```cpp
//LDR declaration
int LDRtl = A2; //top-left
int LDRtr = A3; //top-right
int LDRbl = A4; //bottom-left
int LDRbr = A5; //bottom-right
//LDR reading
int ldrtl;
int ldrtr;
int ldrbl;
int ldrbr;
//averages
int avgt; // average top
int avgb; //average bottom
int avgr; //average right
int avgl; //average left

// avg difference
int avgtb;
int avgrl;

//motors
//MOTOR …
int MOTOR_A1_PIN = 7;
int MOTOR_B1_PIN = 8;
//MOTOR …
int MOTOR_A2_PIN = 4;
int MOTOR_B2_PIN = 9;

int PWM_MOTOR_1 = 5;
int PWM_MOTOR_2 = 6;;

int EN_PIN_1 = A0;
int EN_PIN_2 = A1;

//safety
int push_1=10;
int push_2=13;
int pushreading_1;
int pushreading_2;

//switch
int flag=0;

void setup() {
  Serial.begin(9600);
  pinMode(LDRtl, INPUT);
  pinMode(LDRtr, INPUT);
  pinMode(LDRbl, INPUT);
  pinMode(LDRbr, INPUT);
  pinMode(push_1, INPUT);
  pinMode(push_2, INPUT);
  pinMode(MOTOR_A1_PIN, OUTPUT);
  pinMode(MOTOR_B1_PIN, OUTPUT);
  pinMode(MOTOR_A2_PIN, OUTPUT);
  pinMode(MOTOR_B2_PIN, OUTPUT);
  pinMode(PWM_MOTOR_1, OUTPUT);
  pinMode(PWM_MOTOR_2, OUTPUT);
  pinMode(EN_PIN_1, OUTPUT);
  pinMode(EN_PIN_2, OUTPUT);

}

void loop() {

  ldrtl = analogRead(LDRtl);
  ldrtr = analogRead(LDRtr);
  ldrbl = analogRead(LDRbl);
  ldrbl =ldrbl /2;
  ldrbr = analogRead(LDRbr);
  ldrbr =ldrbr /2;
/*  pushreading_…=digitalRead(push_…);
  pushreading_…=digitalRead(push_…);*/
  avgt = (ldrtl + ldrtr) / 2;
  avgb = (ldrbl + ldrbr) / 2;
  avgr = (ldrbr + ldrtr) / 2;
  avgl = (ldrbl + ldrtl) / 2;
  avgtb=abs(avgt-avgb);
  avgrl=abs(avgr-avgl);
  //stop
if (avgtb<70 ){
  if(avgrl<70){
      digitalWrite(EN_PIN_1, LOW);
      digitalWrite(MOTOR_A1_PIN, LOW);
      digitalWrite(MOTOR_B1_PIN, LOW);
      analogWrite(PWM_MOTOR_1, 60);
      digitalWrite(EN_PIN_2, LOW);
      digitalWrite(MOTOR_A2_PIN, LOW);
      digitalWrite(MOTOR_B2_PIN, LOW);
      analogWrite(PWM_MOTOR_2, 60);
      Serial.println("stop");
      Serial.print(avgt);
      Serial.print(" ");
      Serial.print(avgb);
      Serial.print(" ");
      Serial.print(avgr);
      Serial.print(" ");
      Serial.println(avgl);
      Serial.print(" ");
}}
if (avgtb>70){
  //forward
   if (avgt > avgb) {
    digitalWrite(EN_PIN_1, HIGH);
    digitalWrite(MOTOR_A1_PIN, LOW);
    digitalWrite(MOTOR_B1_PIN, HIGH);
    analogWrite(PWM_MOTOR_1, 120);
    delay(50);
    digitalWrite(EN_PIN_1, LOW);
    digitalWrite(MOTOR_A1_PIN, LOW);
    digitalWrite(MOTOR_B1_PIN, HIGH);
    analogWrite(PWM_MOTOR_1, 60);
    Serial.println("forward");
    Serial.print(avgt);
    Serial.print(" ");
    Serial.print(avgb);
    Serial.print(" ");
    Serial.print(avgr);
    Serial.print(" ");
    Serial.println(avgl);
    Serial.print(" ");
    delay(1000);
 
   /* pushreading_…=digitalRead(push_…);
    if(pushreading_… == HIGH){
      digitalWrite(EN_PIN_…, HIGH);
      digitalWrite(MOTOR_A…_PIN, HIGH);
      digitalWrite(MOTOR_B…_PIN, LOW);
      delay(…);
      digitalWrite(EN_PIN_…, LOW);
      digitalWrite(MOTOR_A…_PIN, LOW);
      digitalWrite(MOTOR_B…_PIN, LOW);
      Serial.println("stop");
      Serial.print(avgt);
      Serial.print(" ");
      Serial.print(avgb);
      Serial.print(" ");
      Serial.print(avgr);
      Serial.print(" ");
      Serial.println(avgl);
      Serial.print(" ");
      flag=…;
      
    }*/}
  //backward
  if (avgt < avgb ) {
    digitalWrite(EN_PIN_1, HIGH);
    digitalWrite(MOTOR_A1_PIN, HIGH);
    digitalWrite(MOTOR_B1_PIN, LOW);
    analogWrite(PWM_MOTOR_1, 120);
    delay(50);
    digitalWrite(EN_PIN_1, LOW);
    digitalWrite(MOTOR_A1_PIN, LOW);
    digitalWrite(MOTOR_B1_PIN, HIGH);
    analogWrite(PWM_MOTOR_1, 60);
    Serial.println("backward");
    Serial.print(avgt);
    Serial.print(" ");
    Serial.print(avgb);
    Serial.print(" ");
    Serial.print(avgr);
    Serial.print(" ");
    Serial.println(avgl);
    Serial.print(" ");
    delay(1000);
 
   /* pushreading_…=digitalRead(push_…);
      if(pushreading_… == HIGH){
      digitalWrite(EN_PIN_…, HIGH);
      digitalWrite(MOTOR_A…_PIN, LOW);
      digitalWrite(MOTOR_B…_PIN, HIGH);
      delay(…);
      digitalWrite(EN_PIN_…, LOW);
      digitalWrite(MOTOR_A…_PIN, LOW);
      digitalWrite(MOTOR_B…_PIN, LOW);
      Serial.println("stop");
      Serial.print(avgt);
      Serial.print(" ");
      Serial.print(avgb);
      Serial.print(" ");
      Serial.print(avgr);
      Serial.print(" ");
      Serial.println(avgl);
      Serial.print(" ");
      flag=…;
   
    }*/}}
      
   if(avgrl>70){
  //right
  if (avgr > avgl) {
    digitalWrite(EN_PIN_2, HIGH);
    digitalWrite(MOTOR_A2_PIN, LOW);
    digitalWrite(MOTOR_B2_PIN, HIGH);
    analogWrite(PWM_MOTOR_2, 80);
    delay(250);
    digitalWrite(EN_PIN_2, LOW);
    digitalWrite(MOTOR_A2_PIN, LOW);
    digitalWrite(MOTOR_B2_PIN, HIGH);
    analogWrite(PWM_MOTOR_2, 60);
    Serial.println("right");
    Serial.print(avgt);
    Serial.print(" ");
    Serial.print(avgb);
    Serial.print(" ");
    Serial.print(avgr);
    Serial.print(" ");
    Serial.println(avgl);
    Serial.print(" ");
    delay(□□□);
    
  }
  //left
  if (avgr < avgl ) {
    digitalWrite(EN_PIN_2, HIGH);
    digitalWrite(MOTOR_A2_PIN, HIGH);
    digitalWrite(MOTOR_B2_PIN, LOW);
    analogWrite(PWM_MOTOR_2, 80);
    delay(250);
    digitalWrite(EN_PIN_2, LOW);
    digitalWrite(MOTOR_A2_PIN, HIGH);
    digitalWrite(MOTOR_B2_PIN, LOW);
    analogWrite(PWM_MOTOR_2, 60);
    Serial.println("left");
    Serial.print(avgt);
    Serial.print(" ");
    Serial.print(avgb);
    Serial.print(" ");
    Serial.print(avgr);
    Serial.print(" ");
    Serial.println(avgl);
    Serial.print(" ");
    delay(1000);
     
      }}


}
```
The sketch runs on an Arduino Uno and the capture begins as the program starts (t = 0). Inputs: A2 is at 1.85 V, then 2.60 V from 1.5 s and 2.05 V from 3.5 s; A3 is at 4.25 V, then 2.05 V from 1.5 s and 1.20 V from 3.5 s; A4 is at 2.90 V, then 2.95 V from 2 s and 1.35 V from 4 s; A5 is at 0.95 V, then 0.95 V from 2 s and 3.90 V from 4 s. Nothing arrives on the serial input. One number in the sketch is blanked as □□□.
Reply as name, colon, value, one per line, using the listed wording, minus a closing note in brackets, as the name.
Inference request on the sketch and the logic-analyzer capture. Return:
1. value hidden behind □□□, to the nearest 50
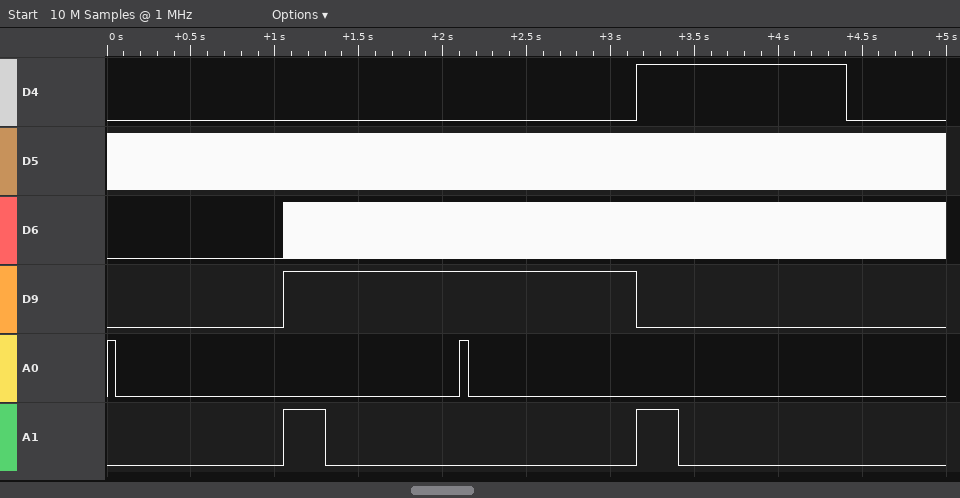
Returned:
value hidden behind □□□, to the nearest 50: 800
